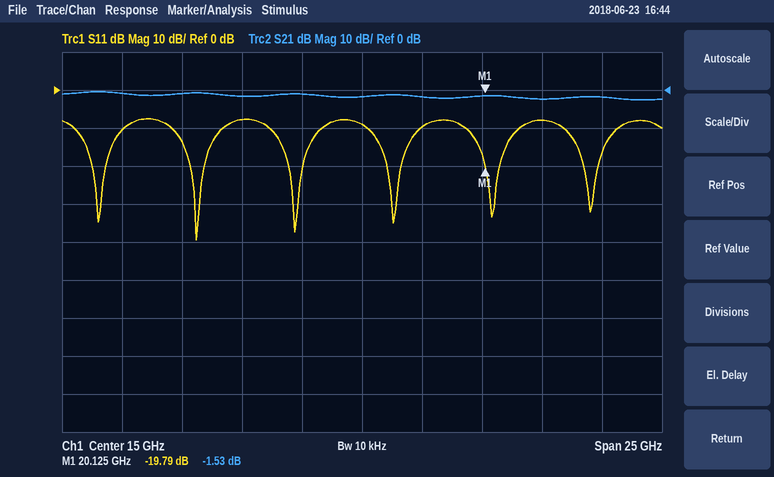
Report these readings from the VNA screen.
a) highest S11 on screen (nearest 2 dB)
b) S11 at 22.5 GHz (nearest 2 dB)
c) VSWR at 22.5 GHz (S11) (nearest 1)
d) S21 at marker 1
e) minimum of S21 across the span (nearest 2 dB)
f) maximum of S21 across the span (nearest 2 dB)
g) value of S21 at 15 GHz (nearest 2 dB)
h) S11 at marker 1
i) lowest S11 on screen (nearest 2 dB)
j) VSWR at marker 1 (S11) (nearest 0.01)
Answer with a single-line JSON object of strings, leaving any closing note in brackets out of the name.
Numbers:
{"highest S11 on screen": "-8 dB", "S11 at 22.5 GHz": "-8 dB", "VSWR at 22.5 GHz (S11)": "2", "S21 at marker 1": "-1.53 dB", "minimum of S21 across the span": "-2 dB", "maximum of S21 across the span": "0 dB", "value of S21 at 15 GHz": "-2 dB", "S11 at marker 1": "-19.79 dB", "lowest S11 on screen": "-40 dB", "VSWR at marker 1 (S11)": "1.23"}
